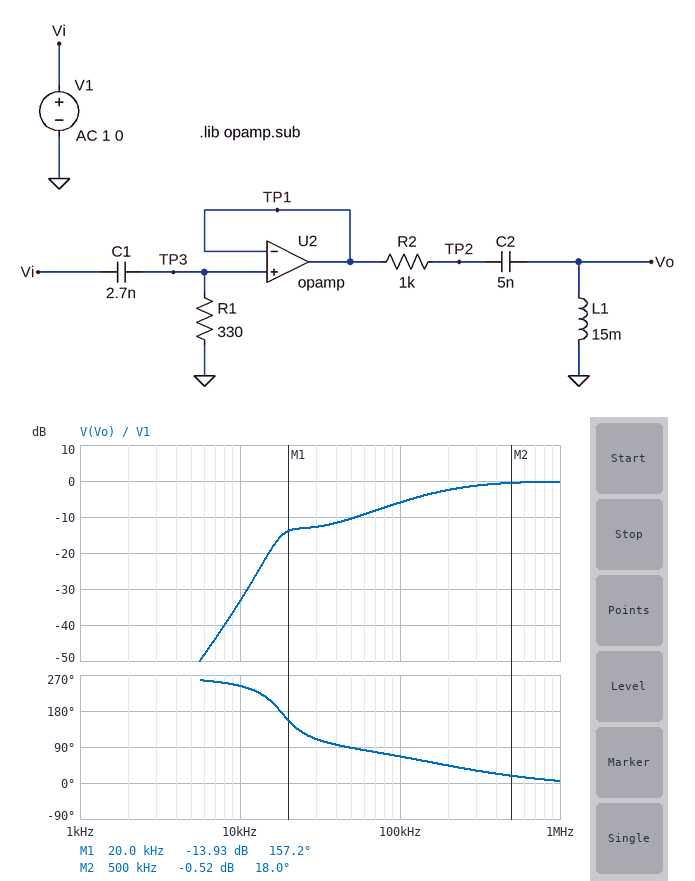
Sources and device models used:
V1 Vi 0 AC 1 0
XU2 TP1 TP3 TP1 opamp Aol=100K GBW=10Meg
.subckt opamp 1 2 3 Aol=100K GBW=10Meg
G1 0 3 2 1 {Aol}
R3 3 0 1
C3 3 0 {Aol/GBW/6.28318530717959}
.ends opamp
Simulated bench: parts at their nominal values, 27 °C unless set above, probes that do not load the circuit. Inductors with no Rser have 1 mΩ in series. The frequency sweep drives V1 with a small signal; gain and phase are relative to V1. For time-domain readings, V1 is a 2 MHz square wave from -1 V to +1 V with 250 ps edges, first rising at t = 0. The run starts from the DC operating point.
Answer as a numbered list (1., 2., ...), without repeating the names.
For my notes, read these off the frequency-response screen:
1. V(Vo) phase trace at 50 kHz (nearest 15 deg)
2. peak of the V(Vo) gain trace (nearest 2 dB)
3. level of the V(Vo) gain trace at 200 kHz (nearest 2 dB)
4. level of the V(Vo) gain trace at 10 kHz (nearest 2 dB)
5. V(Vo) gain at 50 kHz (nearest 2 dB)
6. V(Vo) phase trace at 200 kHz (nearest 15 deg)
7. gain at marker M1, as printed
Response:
1. 90 deg
2. 0 dB
3. -2 dB
4. -34 dB
5. -10 dB
6. 45 deg
7. -13.93 dB
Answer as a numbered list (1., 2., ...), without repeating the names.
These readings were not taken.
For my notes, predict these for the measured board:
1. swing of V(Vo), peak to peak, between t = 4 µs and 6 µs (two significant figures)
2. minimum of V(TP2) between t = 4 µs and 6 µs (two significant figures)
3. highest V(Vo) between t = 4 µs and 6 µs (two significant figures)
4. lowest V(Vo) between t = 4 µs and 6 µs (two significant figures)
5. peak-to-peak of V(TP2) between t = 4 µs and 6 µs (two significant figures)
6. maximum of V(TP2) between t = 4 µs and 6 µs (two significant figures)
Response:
1. 2.1 V
2. -1.1 V
3. 980 mV
4. -1.1 V
5. 2.1 V
6. 1.0 V
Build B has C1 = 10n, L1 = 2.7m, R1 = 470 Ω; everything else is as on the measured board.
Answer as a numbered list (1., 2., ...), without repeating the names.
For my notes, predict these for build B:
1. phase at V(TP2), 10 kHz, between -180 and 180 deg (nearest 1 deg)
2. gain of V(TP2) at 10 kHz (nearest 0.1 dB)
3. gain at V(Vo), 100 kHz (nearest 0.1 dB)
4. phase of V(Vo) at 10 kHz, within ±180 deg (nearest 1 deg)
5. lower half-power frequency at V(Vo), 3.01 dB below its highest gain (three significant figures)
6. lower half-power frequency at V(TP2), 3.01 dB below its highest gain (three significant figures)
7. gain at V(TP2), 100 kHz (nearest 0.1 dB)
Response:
1. 55 deg
2. -11.4 dB
3. -0.5 dB
4. -125 deg
5. 51.3 kHz
6. 88.5 kHz
7. -2.3 dB
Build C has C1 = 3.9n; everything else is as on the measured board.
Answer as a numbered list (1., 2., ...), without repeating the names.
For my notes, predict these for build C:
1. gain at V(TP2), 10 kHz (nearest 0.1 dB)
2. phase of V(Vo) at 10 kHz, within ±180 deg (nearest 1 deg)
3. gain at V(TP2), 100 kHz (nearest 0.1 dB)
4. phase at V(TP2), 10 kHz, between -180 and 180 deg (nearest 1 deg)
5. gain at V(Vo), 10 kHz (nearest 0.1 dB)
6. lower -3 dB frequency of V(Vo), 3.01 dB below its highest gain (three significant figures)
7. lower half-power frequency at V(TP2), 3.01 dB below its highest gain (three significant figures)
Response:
1. -22.7 dB
2. -119 deg
3. -4.1 dB
4. 61 deg
5. -30.2 dB
6. 116 kHz
7. 122 kHz
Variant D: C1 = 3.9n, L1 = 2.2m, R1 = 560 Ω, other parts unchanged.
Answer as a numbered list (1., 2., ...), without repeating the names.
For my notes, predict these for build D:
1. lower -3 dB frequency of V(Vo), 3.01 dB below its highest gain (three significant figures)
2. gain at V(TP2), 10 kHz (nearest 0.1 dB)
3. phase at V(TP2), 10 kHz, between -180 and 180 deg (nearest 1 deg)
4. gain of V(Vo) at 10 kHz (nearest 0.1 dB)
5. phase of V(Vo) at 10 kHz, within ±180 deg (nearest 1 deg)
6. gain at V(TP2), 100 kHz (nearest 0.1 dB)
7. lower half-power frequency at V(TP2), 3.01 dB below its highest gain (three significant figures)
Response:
1. 86.0 kHz
2. -17.8 dB
3. 64 deg
4. -44.6 dB
5. -116 deg
6. -4.6 dB
7. 121 kHz
